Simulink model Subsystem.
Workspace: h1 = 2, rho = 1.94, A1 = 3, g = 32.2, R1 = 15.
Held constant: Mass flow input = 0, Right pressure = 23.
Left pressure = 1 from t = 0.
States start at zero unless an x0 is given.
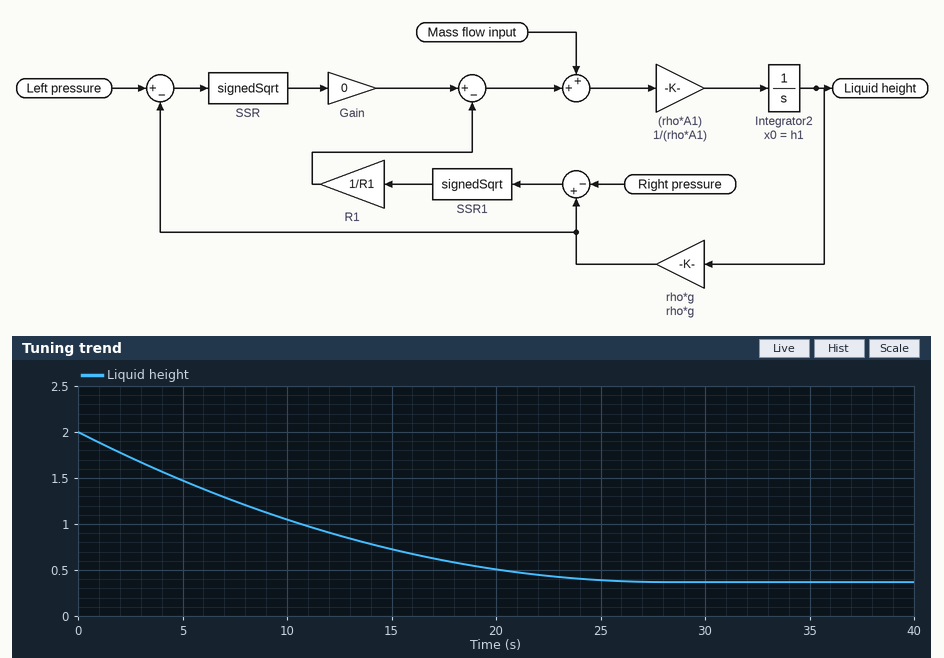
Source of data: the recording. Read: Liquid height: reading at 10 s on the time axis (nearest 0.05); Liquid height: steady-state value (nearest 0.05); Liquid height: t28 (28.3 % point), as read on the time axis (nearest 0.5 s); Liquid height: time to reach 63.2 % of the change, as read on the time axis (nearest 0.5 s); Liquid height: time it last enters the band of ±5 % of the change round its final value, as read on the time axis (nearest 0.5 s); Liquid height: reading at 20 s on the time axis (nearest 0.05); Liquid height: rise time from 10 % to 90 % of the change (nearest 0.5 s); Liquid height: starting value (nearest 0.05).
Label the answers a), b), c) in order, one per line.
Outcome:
a) 1.05
b) 0.35
c) 4.5 s
d) 11.0 s
e) 22.0 s
f) 0.50
g) 18.0 s
h) 2.00
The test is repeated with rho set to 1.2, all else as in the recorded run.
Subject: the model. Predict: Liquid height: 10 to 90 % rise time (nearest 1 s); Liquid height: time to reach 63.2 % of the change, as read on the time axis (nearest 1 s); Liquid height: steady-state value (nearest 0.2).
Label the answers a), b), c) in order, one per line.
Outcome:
a) 13 s
b) 8 s
c) 0.6
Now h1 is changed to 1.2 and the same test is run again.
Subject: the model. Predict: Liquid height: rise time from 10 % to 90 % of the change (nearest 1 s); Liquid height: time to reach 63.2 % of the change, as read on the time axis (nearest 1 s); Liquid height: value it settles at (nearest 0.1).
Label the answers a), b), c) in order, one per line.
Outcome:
a) 13 s
b) 8 s
c) 0.4
